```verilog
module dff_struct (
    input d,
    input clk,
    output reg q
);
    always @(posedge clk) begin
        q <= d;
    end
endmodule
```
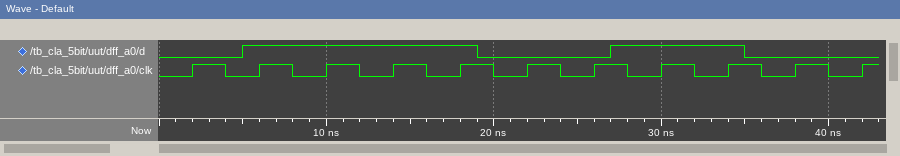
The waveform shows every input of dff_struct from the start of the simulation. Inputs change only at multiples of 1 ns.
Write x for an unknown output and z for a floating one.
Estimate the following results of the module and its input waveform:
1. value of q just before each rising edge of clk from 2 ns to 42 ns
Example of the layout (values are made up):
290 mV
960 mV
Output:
x 0 1 1 1 1 0 0 1 1 0
